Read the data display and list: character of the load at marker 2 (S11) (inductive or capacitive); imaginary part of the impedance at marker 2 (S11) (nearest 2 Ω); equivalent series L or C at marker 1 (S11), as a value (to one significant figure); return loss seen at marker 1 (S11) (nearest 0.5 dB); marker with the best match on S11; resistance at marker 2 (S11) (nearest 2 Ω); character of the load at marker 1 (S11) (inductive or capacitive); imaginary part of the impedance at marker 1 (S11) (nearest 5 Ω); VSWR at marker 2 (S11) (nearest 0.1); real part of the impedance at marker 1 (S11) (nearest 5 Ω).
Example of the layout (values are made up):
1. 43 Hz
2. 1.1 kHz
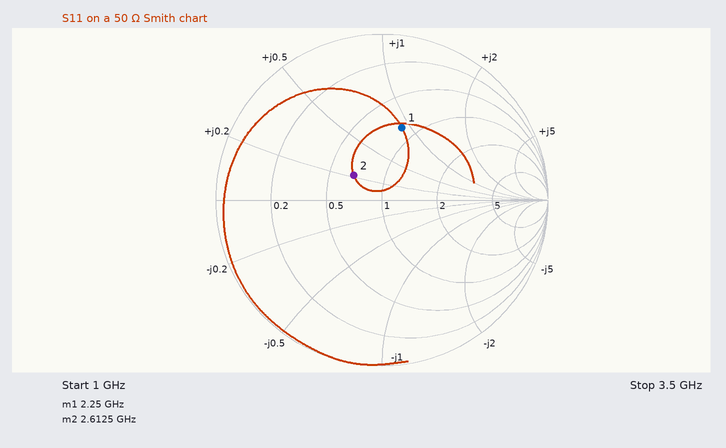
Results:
1. inductive
2. +10 Ω
3. 3 nH
4. 7.0 dB
5. marker 2
6. 34 Ω
7. inductive
8. +45 Ω
9. 1.6
10. 40 Ω
